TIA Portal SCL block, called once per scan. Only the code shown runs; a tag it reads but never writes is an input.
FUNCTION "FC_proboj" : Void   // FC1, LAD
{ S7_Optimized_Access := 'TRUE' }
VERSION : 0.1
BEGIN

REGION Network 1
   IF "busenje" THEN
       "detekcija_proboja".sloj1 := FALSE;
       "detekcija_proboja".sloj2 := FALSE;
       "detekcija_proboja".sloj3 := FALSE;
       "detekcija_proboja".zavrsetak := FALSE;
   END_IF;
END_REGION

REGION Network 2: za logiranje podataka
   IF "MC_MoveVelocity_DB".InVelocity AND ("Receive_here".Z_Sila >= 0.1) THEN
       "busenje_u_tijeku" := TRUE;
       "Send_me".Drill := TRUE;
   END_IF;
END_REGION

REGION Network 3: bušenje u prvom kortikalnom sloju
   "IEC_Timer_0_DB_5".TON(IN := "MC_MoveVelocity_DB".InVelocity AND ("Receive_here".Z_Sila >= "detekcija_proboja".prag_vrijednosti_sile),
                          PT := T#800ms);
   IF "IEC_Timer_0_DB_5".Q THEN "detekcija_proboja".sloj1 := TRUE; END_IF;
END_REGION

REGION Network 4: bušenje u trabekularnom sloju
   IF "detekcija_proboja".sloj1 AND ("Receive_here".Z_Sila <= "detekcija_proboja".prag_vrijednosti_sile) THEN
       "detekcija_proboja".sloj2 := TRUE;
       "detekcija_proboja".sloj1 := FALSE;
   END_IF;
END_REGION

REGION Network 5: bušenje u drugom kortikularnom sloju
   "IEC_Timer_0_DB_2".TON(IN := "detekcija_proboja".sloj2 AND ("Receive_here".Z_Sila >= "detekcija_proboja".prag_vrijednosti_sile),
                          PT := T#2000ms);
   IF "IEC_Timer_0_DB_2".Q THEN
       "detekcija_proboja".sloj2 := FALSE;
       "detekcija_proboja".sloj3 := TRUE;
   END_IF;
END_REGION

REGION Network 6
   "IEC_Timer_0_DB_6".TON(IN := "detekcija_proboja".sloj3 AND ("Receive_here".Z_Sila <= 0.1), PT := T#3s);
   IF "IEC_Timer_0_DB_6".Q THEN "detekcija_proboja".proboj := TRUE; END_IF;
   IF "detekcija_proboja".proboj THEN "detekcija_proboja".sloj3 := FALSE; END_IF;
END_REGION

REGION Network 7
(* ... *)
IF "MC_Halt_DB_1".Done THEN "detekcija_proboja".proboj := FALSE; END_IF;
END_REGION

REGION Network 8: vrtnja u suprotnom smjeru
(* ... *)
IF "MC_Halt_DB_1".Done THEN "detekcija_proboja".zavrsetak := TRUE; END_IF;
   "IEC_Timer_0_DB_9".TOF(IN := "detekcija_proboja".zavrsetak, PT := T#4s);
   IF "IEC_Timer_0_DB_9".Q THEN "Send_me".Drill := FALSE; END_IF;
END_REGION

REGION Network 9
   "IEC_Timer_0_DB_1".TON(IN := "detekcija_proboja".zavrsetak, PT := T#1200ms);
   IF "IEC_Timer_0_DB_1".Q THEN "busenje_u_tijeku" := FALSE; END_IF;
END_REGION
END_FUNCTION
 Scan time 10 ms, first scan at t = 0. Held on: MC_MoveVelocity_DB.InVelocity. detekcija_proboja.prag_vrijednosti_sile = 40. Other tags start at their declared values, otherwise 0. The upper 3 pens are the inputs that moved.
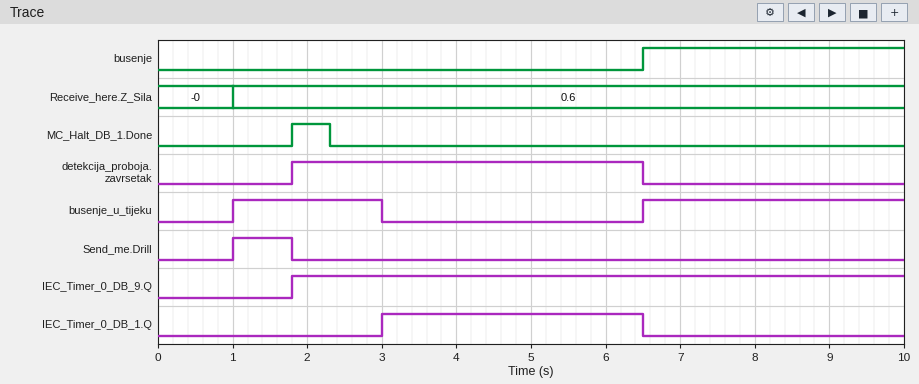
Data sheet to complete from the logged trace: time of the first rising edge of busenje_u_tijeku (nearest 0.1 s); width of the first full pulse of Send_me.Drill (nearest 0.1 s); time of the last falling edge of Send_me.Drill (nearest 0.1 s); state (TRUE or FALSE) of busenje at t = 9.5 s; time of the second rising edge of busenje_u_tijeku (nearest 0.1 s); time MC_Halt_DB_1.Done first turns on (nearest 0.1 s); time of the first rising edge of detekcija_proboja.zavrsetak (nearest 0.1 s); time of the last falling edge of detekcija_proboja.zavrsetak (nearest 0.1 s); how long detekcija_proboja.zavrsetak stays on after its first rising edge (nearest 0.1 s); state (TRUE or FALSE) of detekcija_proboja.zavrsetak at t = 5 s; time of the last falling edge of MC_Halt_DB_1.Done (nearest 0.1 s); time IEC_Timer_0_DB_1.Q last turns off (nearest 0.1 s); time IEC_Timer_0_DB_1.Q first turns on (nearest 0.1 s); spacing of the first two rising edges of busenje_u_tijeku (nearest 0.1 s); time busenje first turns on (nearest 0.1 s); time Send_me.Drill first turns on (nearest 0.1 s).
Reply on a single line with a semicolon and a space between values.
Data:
1.0 s; 0.8 s; 1.8 s; TRUE; 6.5 s; 1.8 s; 1.8 s; 6.5 s; 4.7 s; TRUE; 2.3 s; 6.5 s; 3.0 s; 5.5 s; 6.5 s; 1.0 s
